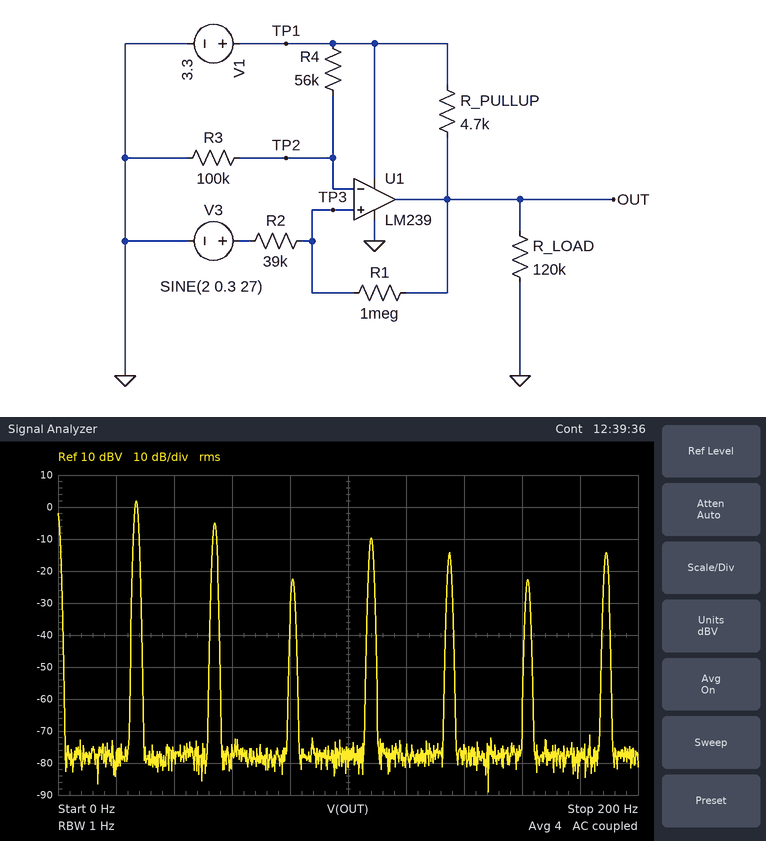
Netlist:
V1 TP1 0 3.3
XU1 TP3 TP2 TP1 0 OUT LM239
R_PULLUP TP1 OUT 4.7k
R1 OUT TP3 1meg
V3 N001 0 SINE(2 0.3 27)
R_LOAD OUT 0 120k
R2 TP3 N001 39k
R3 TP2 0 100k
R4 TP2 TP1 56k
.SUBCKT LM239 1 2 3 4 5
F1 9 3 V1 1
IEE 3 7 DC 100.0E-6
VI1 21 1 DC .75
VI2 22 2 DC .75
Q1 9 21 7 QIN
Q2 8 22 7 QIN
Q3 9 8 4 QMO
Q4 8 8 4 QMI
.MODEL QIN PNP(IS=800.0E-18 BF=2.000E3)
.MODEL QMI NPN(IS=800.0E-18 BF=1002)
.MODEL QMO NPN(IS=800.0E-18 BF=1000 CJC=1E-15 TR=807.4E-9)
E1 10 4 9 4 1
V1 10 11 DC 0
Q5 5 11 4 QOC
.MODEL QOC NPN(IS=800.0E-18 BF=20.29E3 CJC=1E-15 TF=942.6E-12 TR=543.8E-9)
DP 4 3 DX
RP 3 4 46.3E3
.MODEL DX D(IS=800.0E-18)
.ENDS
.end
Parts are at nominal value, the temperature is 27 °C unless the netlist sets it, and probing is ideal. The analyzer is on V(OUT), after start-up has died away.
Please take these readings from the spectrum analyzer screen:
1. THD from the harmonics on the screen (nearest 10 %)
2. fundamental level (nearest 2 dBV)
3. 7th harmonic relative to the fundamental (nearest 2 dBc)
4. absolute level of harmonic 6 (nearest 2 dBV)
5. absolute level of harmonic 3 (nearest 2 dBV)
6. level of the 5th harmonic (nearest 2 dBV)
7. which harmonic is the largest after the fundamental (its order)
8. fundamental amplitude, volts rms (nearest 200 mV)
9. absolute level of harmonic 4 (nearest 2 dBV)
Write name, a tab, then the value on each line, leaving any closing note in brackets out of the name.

THD from the harmonics on the screen	60 %
fundamental level	2 dBV
7th harmonic relative to the fundamental	-16 dBc
absolute level of harmonic 6	-22 dBV
absolute level of harmonic 3	-22 dBV
level of the 5th harmonic	-14 dBV
which harmonic is the largest after the fundamental	2
fundamental amplitude, volts rms	1.2 V
absolute level of harmonic 4	-10 dBV
